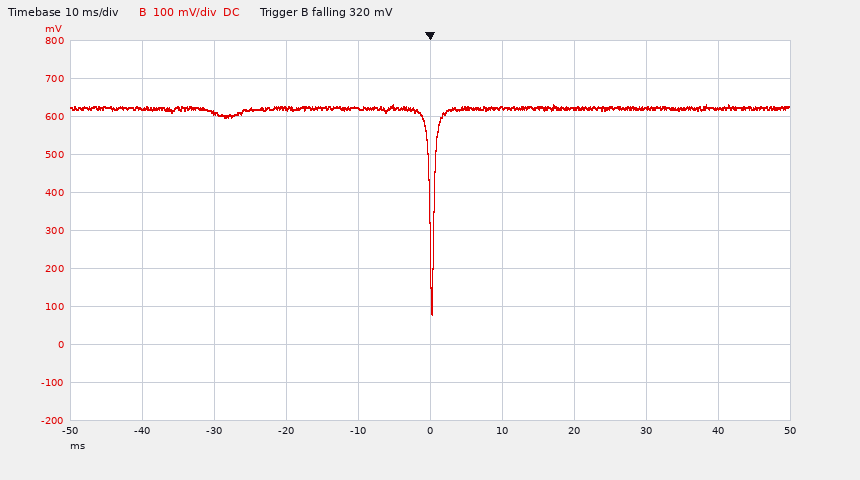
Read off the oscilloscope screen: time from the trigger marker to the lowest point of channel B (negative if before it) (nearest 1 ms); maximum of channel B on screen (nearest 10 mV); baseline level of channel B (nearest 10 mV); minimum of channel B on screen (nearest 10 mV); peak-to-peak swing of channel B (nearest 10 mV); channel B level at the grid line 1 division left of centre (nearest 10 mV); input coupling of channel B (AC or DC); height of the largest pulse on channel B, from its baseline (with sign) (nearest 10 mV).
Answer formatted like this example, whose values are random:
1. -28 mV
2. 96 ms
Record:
1. 0 ms
2. 630 mV
3. 620 mV
4. 80 mV
5. 550 mV
6. 620 mV
7. DC
8. -540 mV
